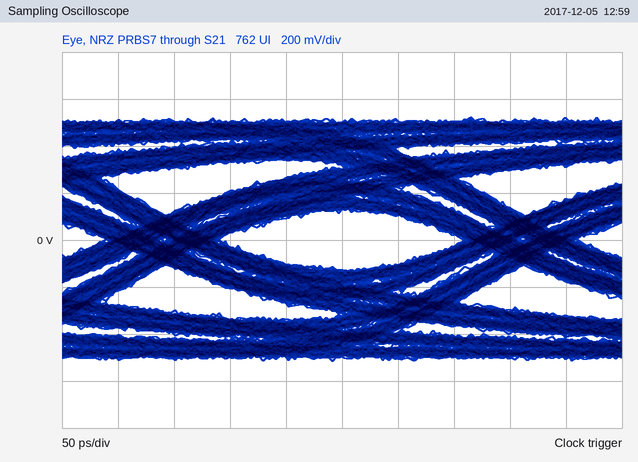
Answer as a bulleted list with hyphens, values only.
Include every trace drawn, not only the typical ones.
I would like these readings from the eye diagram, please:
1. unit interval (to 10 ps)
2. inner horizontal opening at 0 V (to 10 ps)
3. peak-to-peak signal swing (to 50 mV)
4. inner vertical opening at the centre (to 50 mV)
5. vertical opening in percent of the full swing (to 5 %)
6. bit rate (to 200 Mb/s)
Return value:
- 320 ps
- 220 ps
- 1.05 V
- 250 mV
- 25 %
- 3.2 Gb/s
